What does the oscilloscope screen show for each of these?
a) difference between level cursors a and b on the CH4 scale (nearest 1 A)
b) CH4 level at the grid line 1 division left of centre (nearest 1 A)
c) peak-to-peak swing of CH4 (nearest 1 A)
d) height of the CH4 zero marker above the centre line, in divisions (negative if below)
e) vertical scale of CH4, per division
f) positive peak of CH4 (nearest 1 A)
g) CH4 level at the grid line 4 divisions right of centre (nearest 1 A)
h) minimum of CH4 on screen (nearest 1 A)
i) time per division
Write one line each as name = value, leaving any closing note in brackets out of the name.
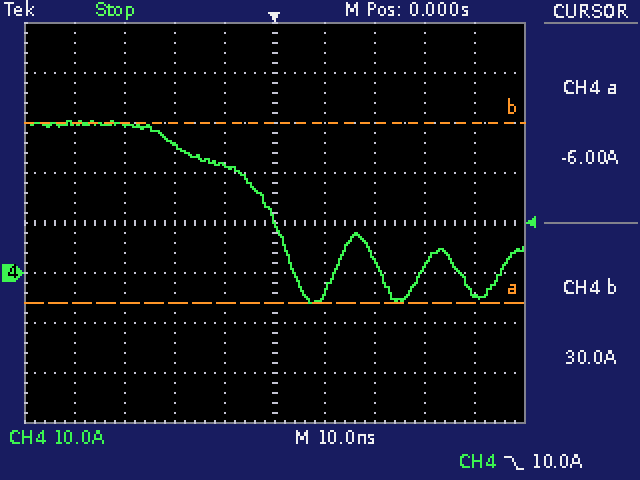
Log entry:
difference between level cursors a and b on the CH4 scale = 36 A
CH4 level at the grid line 1 division left of centre = 22 A
peak-to-peak swing of CH4 = 36 A
height of the CH4 zero marker above the centre line, in divisions = -1.0 div
vertical scale of CH4, per division = 10 A
positive peak of CH4 = 30 A
CH4 level at the grid line 4 divisions right of centre = -4 A
minimum of CH4 on screen = -6 A
time per division = 10 ns
